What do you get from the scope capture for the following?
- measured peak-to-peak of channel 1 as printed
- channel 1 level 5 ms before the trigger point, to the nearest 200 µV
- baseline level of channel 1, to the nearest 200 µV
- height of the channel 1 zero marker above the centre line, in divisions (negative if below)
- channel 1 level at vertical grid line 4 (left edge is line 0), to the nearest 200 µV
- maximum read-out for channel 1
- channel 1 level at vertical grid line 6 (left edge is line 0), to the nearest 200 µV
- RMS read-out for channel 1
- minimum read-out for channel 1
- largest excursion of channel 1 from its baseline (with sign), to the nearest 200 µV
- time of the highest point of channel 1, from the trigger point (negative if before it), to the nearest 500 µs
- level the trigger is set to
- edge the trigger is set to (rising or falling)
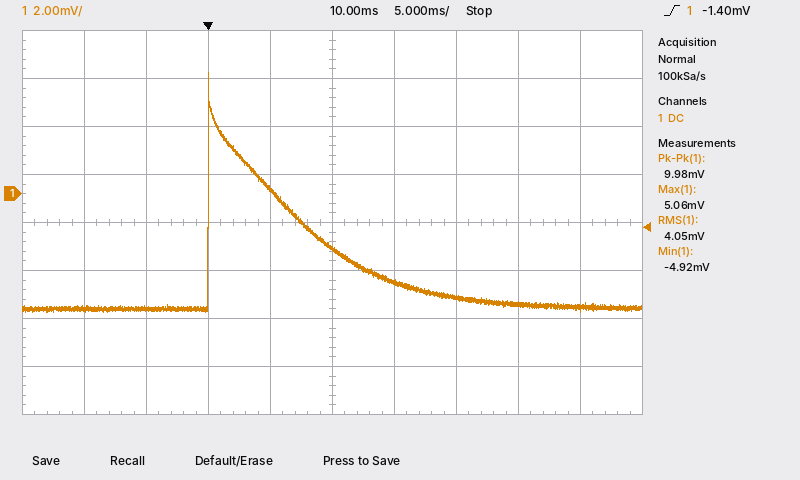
9.98 mV
-4.8 mV
-4.8 mV
+0.6 div
200 µV
5.06 mV
-3.6 mV
4.05 mV
-4.92 mV
+9.8 mV
0.0 ms
-1.40 mV
rising
